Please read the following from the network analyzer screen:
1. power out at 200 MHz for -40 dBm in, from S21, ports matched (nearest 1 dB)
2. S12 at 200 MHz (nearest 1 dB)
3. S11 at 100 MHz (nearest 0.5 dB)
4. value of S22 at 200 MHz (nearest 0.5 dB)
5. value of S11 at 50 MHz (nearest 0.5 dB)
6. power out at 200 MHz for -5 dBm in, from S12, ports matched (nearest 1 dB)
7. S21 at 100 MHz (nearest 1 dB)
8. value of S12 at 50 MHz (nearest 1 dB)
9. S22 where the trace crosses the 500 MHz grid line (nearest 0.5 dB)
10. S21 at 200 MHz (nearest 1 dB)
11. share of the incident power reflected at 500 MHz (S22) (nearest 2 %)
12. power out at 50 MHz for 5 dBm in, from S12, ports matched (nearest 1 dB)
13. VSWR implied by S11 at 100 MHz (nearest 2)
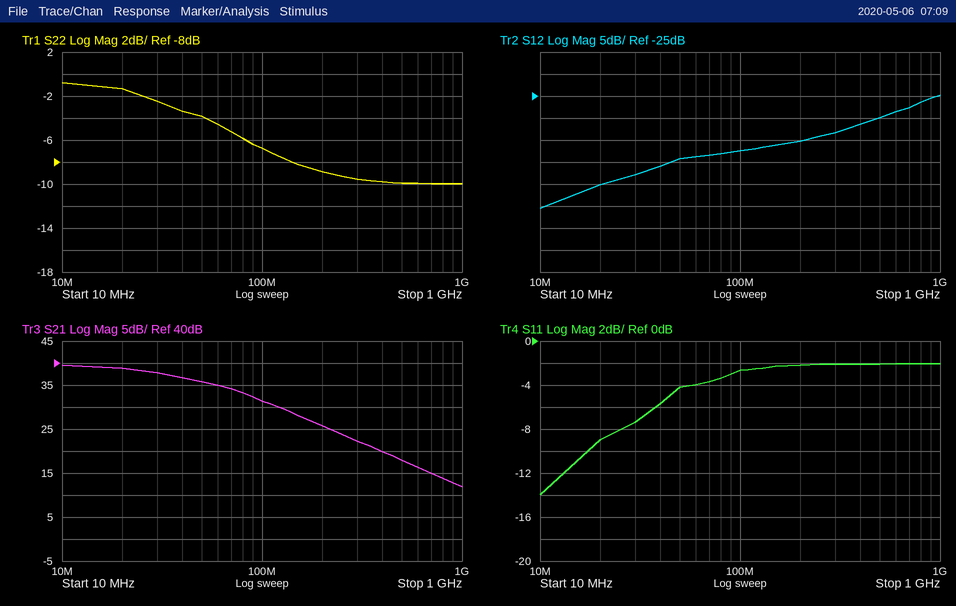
-14 dBm
-35 dB
-2.5 dB
-9.0 dB
-4.0 dB
-40 dBm
31 dB
-39 dB
-10.0 dB
26 dB
10 %
-34 dBm
6
